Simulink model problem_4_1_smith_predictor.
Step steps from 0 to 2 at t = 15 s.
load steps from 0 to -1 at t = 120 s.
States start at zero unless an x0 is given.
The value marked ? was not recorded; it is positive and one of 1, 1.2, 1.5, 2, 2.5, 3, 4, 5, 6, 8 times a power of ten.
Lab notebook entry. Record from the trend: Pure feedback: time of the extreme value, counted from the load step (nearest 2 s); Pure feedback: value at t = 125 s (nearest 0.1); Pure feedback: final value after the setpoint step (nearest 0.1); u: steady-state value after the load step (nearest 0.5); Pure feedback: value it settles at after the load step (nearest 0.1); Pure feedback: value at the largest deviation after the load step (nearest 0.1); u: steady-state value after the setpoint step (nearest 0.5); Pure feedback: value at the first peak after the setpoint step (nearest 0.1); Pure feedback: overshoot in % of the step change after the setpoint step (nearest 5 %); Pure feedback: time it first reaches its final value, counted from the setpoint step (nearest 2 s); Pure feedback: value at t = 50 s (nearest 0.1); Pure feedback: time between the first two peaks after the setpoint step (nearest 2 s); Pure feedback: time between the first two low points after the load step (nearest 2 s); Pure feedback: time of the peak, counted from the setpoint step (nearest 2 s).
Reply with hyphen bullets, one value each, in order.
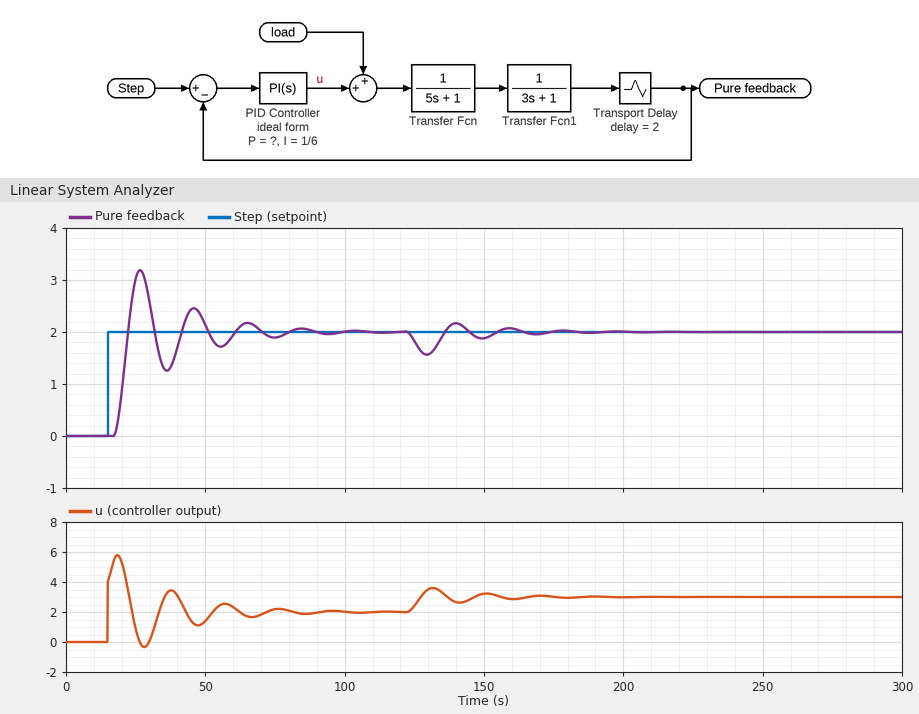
- 10 s
- 1.8
- 2.0
- 3.0
- 2.0
- 1.6
- 2.0
- 3.2
- 60 %
- 8 s
- 2.1
- 20 s
- 20 s
- 12 s
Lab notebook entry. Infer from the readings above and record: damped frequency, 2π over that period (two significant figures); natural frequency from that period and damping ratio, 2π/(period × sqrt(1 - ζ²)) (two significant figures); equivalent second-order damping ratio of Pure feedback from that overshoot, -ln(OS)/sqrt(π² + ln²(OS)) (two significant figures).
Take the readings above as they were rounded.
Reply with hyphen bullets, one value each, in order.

- 0.31 rad/s
- 0.32 rad/s
- 0.16
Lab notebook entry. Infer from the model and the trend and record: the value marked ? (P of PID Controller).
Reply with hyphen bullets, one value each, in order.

- 2
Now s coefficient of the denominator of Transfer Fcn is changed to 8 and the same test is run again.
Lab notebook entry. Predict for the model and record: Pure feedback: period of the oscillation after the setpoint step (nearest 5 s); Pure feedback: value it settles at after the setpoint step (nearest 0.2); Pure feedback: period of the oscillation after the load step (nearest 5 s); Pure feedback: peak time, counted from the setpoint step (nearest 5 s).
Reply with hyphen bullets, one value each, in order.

- 25 s
- 2.0
- 25 s
- 15 s
